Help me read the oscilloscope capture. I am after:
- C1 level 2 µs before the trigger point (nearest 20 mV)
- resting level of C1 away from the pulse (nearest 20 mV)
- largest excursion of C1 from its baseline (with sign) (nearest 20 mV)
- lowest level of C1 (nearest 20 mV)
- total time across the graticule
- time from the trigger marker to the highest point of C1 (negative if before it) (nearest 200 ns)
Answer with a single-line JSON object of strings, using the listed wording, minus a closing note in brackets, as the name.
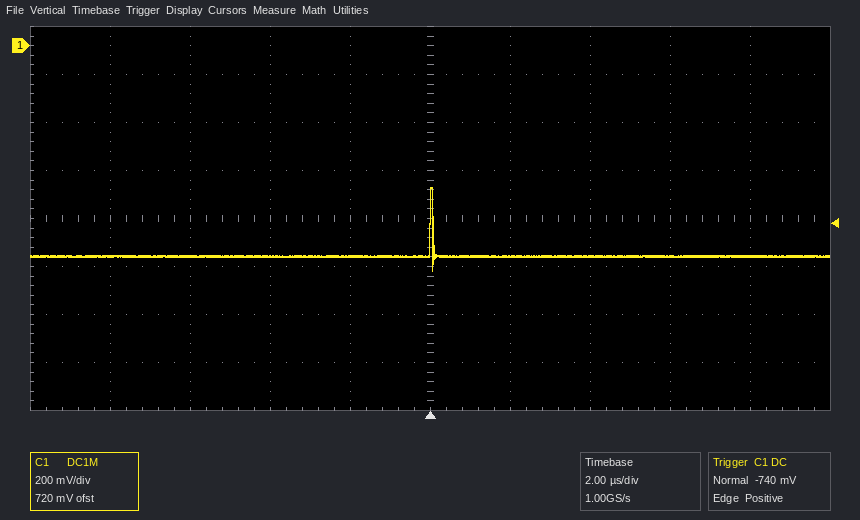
{"C1 level 2 µs before the trigger point": "-880 mV", "resting level of C1 away from the pulse": "-880 mV", "largest excursion of C1 from its baseline (with sign)": "+280 mV", "lowest level of C1": "-940 mV", "total time across the graticule": "20 µs", "time from the trigger marker to the highest point of C1 (negative if before it)": "0.0 µs"}
